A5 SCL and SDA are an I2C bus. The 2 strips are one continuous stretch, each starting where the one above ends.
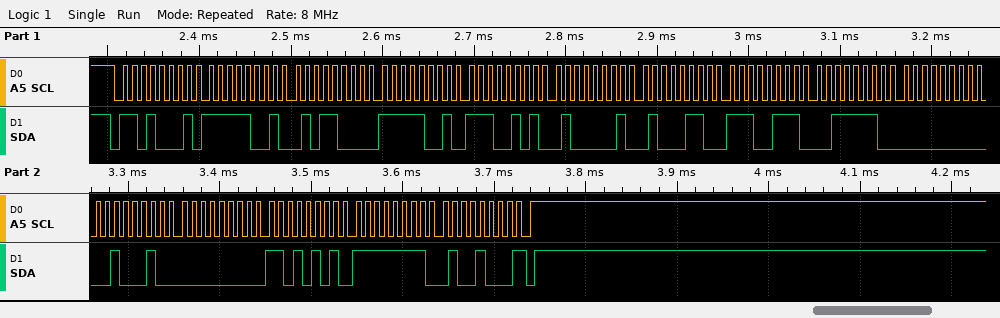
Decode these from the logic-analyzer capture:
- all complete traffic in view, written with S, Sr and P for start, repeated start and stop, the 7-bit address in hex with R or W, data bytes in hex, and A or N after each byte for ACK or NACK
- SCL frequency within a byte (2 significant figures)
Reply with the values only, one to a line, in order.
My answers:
S 68R A F9 A 58 A F9 A E5 A 41 A 46 A E7 A 3E A 00 A 22 A 00 A D5 A FF A 48 N P
100 kHz
